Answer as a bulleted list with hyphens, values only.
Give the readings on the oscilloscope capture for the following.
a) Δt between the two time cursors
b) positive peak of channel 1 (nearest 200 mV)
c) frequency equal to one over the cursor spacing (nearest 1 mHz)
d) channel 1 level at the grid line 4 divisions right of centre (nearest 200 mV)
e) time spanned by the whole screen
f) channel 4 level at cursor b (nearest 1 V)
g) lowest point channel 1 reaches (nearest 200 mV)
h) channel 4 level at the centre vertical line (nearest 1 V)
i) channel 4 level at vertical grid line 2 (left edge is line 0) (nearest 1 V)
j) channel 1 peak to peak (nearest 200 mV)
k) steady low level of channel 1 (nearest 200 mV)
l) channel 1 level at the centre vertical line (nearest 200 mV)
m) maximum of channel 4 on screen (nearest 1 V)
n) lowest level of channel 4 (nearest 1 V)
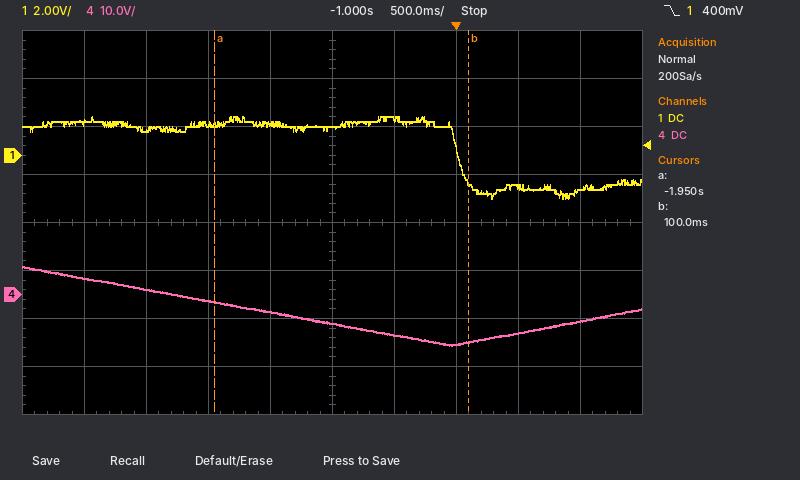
- 2.05 s
- 1.6 V
- 488 mHz
- -1.4 V
- 5 s
- -10 V
- -1.8 V
- -6 V
- 1 V
- 3.4 V
- -1.4 V
- 1.2 V
- 6 V
- -11 V
